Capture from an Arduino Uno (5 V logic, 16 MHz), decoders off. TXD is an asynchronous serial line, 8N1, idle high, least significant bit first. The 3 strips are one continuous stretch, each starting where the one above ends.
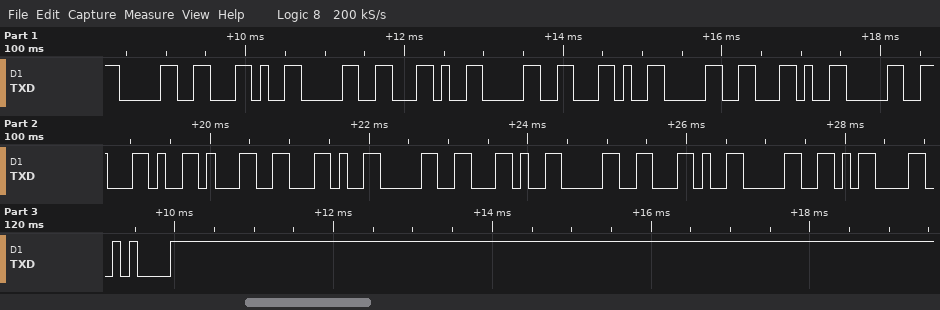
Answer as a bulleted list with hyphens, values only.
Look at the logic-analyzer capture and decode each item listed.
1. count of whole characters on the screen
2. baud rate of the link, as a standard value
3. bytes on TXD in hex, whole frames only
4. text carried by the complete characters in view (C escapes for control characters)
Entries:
- 19
- 9600 baud
- 0x30 0x2C 0x30 0x2C 0x30 0x2C 0x30 0x2C 0x30 0x2C 0x31 0x2C 0x30 0x2C 0x30 0x2C 0x30 0x0D 0x0A
- "0,0,0,0,0,1,0,0,0\r\n"
